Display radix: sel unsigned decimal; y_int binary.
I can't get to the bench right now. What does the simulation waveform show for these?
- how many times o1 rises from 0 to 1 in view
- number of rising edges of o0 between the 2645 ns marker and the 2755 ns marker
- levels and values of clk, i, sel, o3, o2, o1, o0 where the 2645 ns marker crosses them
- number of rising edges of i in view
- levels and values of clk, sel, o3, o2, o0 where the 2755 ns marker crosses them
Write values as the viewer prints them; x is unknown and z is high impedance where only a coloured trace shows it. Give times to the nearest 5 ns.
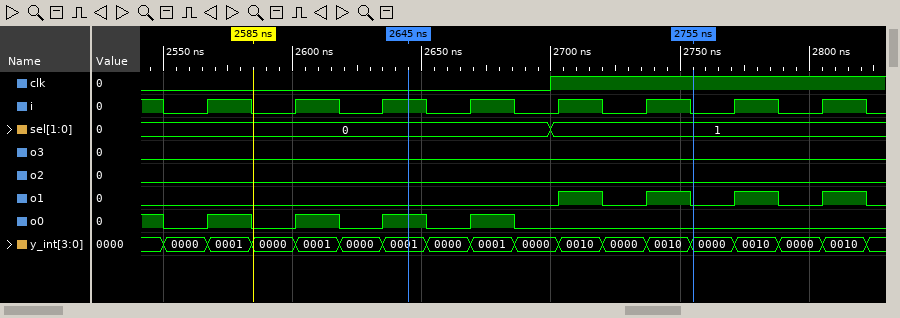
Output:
4
1
clk=0, i=1, sel=0, o3=0, o2=0, o1=0, o0=1
8
clk=1, sel=1, o3=0, o2=0, o0=0
